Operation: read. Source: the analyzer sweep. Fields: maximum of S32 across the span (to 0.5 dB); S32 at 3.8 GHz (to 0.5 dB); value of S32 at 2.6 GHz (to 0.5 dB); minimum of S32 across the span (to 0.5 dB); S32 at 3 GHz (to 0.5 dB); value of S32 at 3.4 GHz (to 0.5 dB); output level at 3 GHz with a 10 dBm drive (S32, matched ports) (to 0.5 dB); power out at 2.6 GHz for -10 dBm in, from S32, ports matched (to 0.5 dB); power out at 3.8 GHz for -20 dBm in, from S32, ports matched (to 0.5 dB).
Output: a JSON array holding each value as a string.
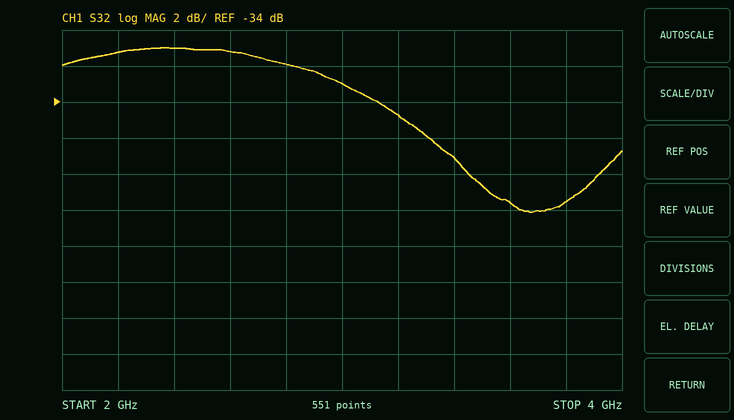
["-31.0 dB", "-39.5 dB", "-31.0 dB", "-40.0 dB", "-33.0 dB", "-37.0 dB", "-23.0 dBm", "-41.0 dBm", "-59.5 dBm"]
